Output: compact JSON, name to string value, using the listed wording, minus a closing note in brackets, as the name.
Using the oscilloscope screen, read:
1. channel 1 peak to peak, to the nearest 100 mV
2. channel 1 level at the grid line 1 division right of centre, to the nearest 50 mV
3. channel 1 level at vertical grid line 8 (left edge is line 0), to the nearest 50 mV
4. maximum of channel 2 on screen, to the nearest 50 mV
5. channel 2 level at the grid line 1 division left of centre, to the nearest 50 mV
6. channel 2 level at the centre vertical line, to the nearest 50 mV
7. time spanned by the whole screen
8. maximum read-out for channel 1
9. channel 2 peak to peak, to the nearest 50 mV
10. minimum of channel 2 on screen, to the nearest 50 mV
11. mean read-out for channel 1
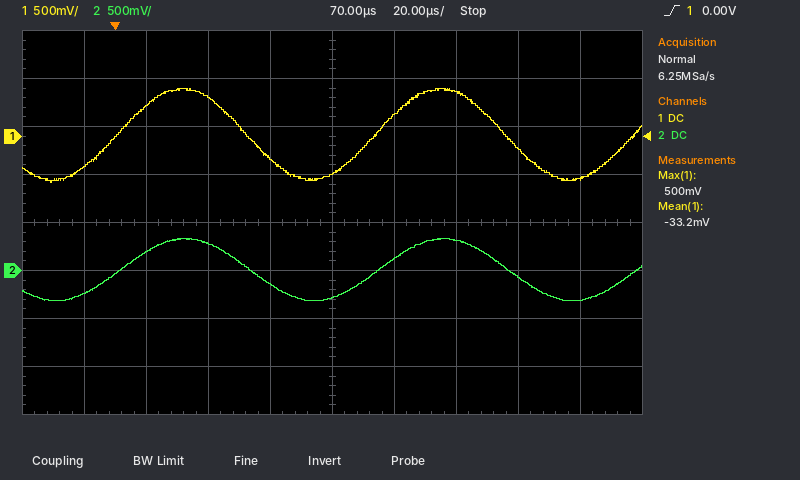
{"channel 1 peak to peak, to the nearest 100 mV": "1.00 V", "channel 1 level at the grid line 1 division right of centre, to the nearest 50 mV": "200 mV", "channel 1 level at vertical grid line 8 (left edge is line 0), to the nearest 50 mV": "-150 mV", "maximum of channel 2 on screen, to the nearest 50 mV": "350 mV", "channel 2 level at the grid line 1 division left of centre, to the nearest 50 mV": "-150 mV", "channel 2 level at the centre vertical line, to the nearest 50 mV": "-300 mV", "time spanned by the whole screen": "200 µs", "maximum read-out for channel 1": "500 mV", "channel 2 peak to peak, to the nearest 50 mV": "650 mV", "minimum of channel 2 on screen, to the nearest 50 mV": "-300 mV", "mean read-out for channel 1": "-33.2 mV"}
